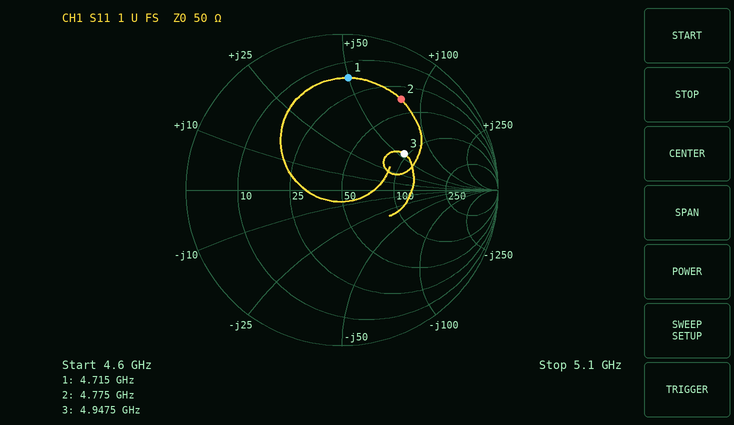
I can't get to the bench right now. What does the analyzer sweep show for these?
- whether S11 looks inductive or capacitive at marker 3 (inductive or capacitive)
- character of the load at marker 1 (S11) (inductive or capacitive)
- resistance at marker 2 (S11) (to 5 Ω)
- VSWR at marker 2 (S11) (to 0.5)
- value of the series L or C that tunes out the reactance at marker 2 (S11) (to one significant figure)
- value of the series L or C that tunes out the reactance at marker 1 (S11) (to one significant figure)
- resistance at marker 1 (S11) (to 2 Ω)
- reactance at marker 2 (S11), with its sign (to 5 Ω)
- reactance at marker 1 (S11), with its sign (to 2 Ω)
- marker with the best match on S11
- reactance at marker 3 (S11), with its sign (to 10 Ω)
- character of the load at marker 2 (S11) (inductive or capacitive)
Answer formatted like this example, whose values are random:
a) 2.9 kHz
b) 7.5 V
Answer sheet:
a) inductive
b) inductive
c) 35 Ω
d) 5.5
e) 400 fF
f) 700 fF
g) 16 Ω
h) +80 Ω
i) +50 Ω
j) marker 3
k) +60 Ω
l) inductive
